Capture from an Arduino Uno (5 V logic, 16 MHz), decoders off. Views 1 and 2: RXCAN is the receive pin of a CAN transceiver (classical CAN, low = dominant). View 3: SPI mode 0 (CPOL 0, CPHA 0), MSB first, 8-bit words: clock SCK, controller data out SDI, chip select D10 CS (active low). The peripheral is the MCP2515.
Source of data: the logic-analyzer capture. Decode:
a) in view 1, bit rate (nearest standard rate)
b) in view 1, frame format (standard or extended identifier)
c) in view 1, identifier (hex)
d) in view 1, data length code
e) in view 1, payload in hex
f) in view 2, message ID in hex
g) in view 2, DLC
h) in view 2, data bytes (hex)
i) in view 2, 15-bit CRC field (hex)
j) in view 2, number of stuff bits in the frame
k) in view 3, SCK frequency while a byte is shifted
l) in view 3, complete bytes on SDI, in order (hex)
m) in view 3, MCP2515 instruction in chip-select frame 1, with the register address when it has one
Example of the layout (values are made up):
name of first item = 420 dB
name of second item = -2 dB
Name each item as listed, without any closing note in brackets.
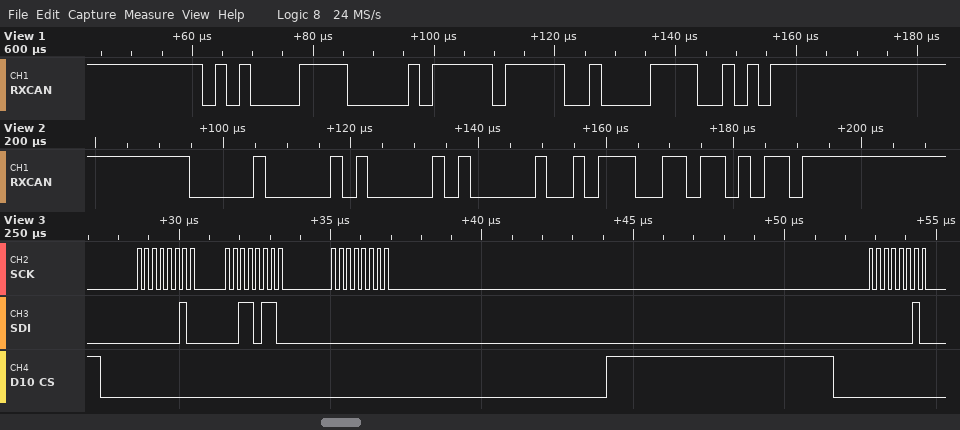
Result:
in view 1, bit rate = 500 kbit/s
in view 1, frame format = standard
in view 1, identifier = 0x50F
in view 1, data length code = 1
in view 1, payload in hex = FF
in view 2, message ID in hex = 0x001
in view 2, DLC = 1
in view 2, data bytes = 01
in view 2, 15-bit CRC field = 0x39B5
in view 2, number of stuff bits in the frame = 4
in view 3, SCK frequency while a byte is shifted = 4 MHz
in view 3, complete bytes on SDI, in order = 0x02 0x36 0x00 0x02
in view 3, MCP2515 instruction in chip-select frame 1, with the register address when it has one = WRITE 0x36
